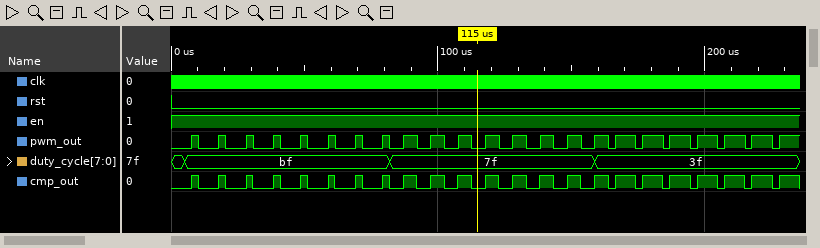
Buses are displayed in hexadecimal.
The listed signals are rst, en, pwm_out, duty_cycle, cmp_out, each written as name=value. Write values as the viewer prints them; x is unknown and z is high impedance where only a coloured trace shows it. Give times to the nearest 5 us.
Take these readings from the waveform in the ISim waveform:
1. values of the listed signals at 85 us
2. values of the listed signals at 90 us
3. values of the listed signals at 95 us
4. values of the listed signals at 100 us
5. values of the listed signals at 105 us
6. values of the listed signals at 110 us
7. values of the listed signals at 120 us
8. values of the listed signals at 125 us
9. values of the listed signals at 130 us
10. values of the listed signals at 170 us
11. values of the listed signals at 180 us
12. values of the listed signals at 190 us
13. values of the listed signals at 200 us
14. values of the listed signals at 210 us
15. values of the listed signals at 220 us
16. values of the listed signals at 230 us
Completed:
rst=0, en=1, pwm_out=0, duty_cycle=7f, cmp_out=0
rst=0, en=1, pwm_out=1, duty_cycle=7f, cmp_out=1
rst=0, en=1, pwm_out=0, duty_cycle=7f, cmp_out=0
rst=0, en=1, pwm_out=1, duty_cycle=7f, cmp_out=1
rst=0, en=1, pwm_out=0, duty_cycle=7f, cmp_out=0
rst=0, en=1, pwm_out=1, duty_cycle=7f, cmp_out=1
rst=0, en=1, pwm_out=1, duty_cycle=7f, cmp_out=1
rst=0, en=1, pwm_out=0, duty_cycle=7f, cmp_out=0
rst=0, en=1, pwm_out=1, duty_cycle=7f, cmp_out=1
rst=0, en=1, pwm_out=1, duty_cycle=3f, cmp_out=1
rst=0, en=1, pwm_out=1, duty_cycle=3f, cmp_out=1
rst=0, en=1, pwm_out=1, duty_cycle=3f, cmp_out=1
rst=0, en=1, pwm_out=1, duty_cycle=3f, cmp_out=1
rst=0, en=1, pwm_out=1, duty_cycle=3f, cmp_out=1
rst=0, en=1, pwm_out=1, duty_cycle=3f, cmp_out=1
rst=0, en=1, pwm_out=1, duty_cycle=3f, cmp_out=1
